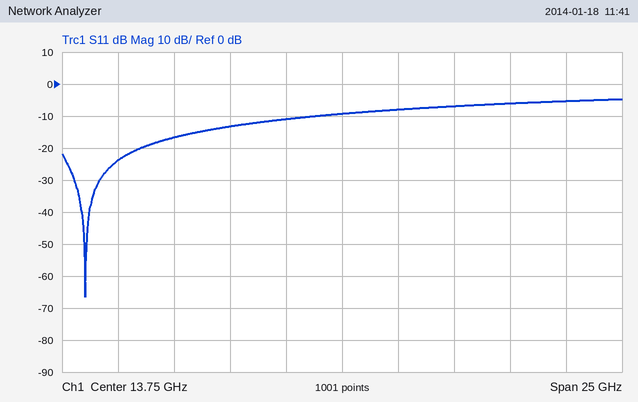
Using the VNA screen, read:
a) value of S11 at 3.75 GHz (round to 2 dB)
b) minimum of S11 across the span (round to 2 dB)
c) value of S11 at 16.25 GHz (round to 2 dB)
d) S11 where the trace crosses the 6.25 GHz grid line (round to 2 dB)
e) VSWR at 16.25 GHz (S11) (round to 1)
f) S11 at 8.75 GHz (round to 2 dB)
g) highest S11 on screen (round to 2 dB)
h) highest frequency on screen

-24 dB
-66 dB
-8 dB
-16 dB
2
-14 dB
-4 dB
26.25 GHz
